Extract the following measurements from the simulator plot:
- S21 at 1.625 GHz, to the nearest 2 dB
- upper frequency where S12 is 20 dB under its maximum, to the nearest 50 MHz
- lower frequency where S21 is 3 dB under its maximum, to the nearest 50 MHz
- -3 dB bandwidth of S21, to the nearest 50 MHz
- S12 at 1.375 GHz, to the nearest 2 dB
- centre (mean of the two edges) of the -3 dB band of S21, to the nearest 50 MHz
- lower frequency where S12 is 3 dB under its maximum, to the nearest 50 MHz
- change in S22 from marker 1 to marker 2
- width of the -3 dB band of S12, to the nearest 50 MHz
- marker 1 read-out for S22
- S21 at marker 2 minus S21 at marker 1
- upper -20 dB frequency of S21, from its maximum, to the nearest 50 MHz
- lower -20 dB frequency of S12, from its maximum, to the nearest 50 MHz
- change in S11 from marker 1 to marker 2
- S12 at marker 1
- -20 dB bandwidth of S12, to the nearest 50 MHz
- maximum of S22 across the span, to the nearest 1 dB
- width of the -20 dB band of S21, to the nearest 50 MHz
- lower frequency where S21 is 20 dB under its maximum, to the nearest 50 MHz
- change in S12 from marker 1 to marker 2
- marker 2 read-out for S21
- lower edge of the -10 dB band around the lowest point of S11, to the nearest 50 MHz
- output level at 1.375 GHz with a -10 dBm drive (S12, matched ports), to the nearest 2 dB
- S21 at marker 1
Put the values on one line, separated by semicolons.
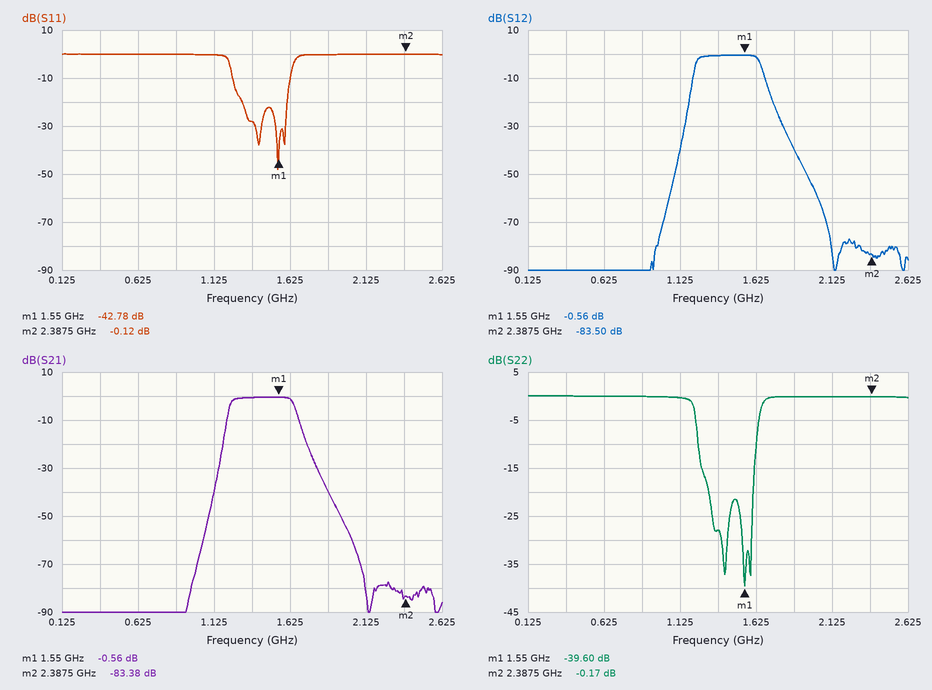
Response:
-2 dB; 1.75 GHz; 1.25 GHz; 400 MHz; 0 dB; 1.45 GHz; 1.25 GHz; 39.43 dB; 400 MHz; -39.60 dB; -82.82 dB; 1.75 GHz; 1.20 GHz; 42.66 dB; -0.56 dB; 550 MHz; 0 dB; 550 MHz; 1.20 GHz; -82.94 dB; -83.38 dB; 1.25 GHz; -10 dBm; -0.56 dB
